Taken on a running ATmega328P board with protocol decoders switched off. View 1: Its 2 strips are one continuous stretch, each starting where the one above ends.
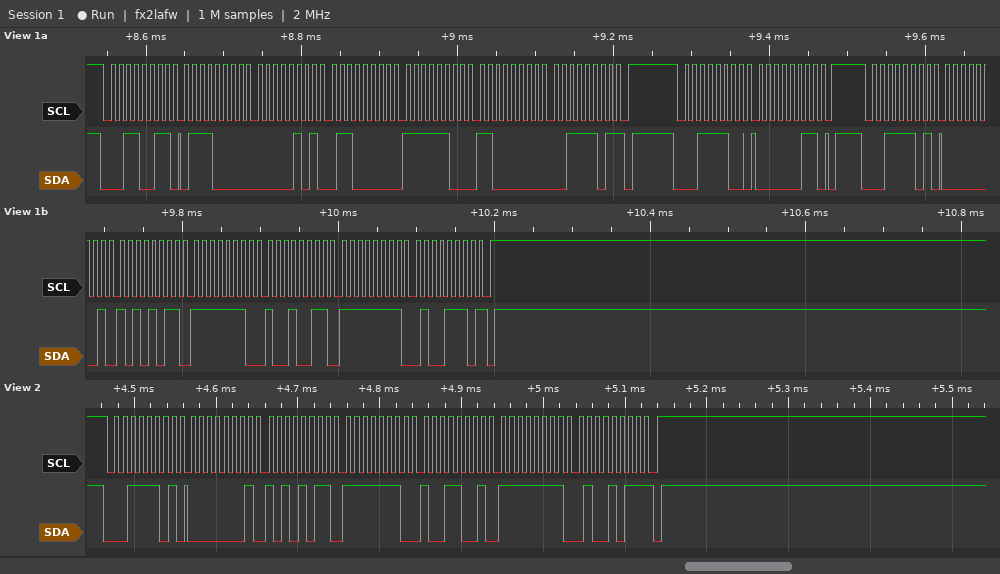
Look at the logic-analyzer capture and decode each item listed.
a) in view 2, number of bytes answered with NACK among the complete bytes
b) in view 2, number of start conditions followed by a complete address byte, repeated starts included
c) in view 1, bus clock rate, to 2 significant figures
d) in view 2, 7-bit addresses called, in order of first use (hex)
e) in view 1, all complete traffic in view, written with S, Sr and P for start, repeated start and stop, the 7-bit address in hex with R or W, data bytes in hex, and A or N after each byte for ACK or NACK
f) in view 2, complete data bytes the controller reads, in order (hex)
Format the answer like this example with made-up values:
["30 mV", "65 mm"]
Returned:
["1", "1", "100 kHz", "0x1E", "S 19R A 70 A 05 A 60 A FC A C0 A 3D N P S 1EW A 03 A P S 1ER A 01 A AB A FE A 93 A FF A 4E N P", "01 AB FE 99 FF 4B"]
